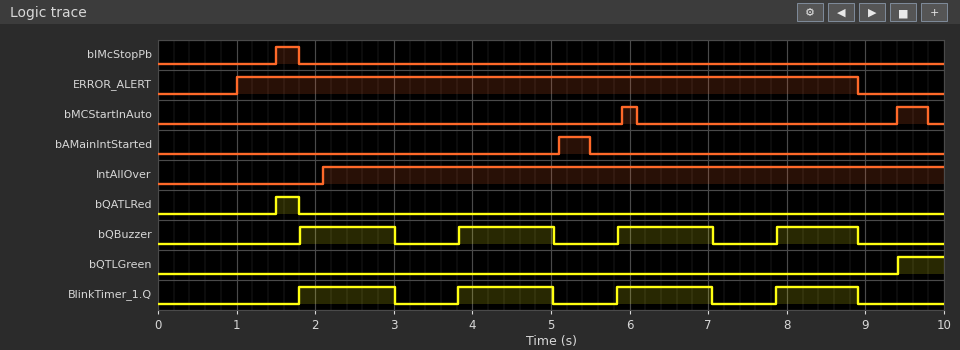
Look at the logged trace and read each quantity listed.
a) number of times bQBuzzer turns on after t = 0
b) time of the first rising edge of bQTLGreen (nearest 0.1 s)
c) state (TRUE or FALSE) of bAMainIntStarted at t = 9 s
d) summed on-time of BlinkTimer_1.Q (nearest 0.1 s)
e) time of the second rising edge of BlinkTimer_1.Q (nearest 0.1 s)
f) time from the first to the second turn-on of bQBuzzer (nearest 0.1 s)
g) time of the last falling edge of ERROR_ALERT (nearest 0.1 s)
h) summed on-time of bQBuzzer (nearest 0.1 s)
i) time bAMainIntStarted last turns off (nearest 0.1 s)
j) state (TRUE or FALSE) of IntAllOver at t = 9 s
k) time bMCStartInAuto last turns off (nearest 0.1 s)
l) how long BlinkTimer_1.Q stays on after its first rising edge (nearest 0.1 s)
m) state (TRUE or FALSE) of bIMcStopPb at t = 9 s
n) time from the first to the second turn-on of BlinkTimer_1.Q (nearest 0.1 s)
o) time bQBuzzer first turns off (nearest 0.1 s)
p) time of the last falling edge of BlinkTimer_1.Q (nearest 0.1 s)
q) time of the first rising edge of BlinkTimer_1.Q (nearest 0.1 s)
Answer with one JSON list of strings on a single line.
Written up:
["4", "9.4 s", "FALSE", "4.7 s", "3.8 s", "2.0 s", "8.9 s", "4.7 s", "5.5 s", "TRUE", "9.8 s", "1.2 s", "FALSE", "2.0 s", "3.0 s", "8.9 s", "1.8 s"]
